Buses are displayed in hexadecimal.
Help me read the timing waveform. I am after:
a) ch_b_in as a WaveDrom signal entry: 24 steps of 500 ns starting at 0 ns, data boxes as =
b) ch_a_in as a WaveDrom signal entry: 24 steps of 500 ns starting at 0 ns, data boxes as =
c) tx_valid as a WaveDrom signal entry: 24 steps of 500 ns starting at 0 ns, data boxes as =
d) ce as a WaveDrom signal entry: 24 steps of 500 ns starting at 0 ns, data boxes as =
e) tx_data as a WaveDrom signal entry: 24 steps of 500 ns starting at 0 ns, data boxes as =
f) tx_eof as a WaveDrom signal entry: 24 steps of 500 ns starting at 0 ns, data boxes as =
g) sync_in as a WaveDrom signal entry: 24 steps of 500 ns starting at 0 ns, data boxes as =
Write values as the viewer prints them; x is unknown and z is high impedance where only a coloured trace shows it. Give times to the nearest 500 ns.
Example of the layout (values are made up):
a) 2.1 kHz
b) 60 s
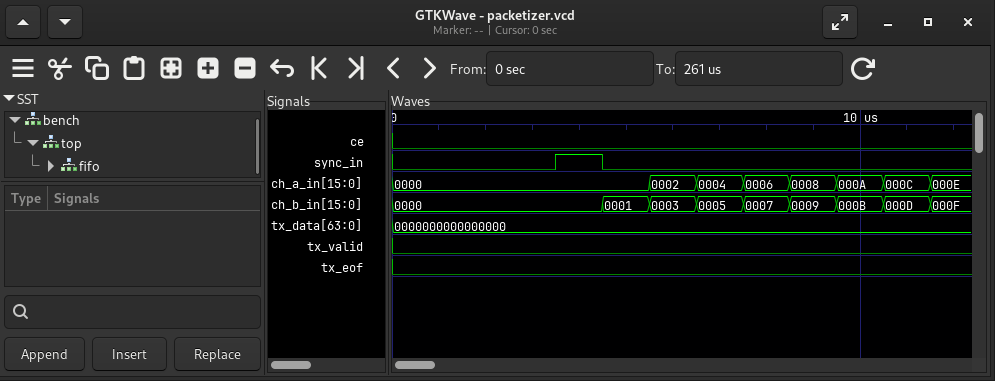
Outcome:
a) {name: 'ch_b_in', wave: '=........=.=.=.=.=.=.=.=', data: '0000 0001 0003 0005 0007 0009 000B 000D 000F'}
b) {name: 'ch_a_in', wave: '=..........=.=.=.=.=.=.=', data: '0000 0002 0004 0006 0008 000A 000C 000E'}
c) {name: 'tx_valid', wave: '0.......................'}
d) {name: 'ce', wave: '0.......................'}
e) {name: 'tx_data', wave: '=.......................', data: '0000000000000000'}
f) {name: 'tx_eof', wave: '0.......................'}
g) {name: 'sync_in', wave: '0......1.0..............'}
